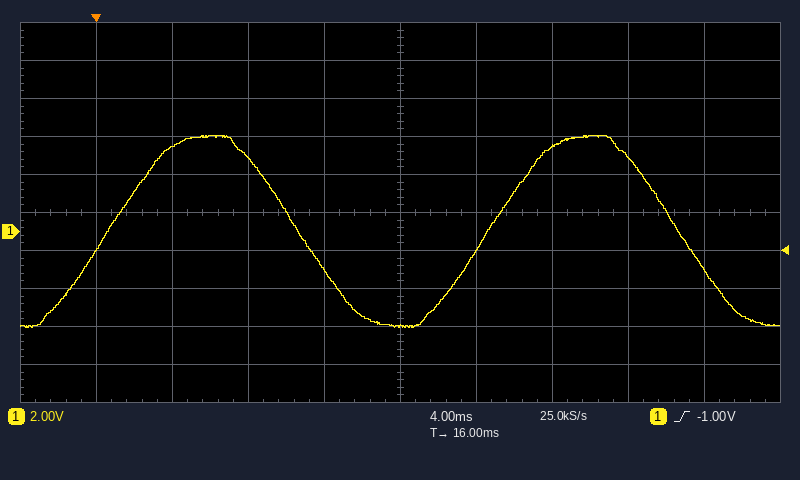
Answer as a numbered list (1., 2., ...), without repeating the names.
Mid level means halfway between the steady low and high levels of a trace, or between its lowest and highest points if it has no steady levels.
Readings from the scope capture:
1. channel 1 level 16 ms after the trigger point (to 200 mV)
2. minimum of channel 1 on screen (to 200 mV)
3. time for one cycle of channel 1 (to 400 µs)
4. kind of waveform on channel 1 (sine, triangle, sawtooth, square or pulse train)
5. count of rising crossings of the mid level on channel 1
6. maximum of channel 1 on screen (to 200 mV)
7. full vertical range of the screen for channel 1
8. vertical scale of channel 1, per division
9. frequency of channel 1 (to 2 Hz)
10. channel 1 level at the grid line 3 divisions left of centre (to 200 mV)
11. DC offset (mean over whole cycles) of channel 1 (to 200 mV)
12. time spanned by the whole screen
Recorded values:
1. -5.0 V
2. -5.0 V
3. 20.0 ms
4. sine
5. 2
6. 5.0 V
7. 20 V
8. 2 V
9. 50 Hz
10. 4.4 V
11. 0.0 V
12. 40 ms
